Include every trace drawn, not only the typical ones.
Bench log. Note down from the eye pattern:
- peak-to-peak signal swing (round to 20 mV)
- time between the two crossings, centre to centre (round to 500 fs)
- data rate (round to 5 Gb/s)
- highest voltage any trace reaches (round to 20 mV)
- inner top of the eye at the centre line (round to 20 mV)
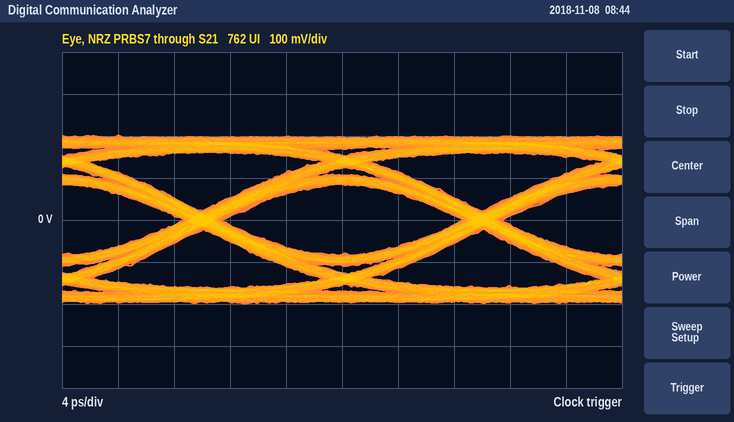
400 mV
20.0 ps
50 Gb/s
200 mV
80 mV
